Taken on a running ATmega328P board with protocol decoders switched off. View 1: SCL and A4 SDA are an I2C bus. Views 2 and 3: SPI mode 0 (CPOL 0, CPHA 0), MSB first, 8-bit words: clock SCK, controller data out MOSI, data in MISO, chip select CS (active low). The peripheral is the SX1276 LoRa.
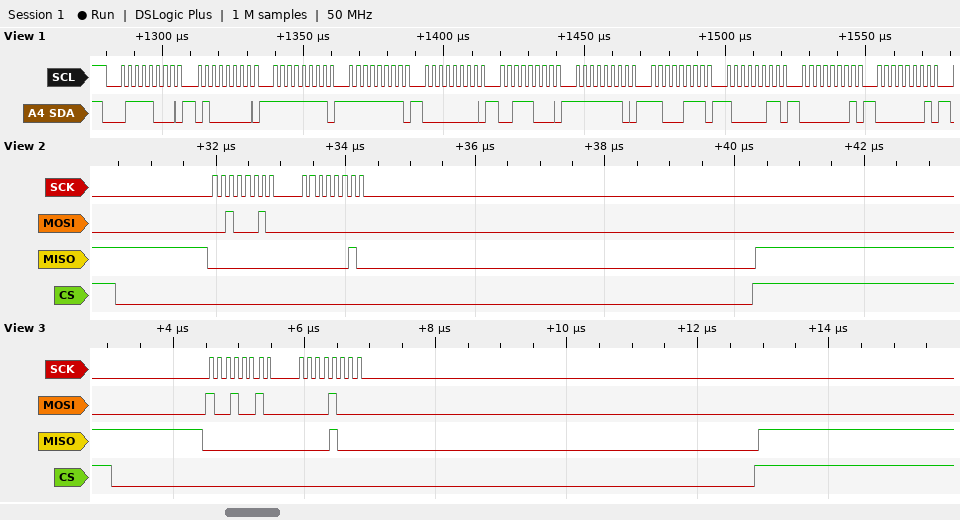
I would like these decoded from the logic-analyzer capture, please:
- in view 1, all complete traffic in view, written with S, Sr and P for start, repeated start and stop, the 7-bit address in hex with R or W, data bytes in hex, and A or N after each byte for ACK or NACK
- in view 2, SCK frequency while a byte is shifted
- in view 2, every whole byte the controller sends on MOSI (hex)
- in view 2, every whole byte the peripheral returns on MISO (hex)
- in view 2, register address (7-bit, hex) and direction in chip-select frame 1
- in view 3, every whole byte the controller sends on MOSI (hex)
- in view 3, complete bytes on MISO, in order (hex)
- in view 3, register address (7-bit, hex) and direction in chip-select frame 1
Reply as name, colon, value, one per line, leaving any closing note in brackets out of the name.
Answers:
in view 1, all complete traffic in view, written with S, Sr and P for start, repeated start and stop, the 7-bit address in hex with R or W, data bytes in hex, and A or N after each byte for ACK or NACK: S 3CW A 40 A FF A FF A 00 A 38 A FE A C7 A 83 A 01 A 01 A
in view 2, SCK frequency while a byte is shifted: 8 MHz
in view 2, every whole byte the controller sends on MOSI: 22 00
in view 2, every whole byte the peripheral returns on MISO: 00 02
in view 2, register address (7-bit, hex) and direction in chip-select frame 1: 0x22 read
in view 3, every whole byte the controller sends on MOSI: 92 08
in view 3, complete bytes on MISO, in order: 00 08
in view 3, register address (7-bit, hex) and direction in chip-select frame 1: 0x12 write
